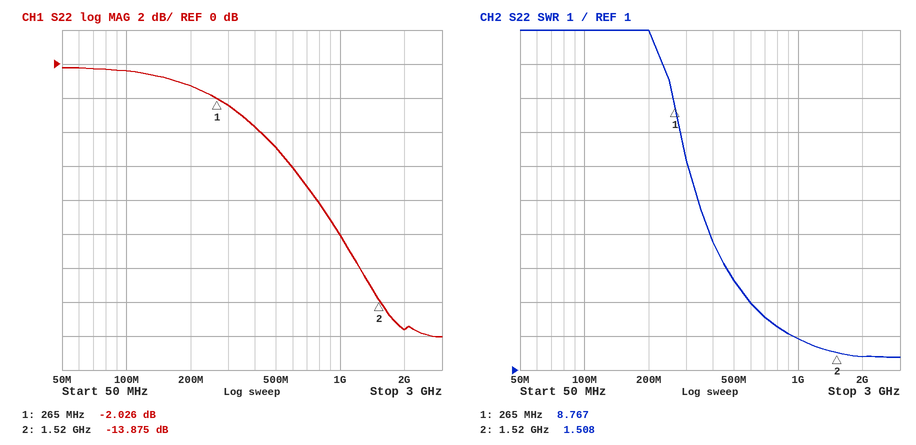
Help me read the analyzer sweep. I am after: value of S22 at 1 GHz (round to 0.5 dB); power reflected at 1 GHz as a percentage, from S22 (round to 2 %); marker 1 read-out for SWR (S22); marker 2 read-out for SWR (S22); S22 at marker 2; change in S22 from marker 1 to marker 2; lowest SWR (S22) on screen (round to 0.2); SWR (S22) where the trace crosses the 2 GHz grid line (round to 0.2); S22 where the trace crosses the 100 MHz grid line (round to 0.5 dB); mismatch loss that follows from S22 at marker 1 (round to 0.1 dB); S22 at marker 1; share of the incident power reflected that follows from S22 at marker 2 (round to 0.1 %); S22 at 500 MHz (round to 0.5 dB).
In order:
-10.0 dB
10 %
8.767
1.508
-13.875 dB
-11.849 dB
1.4
1.4
-0.5 dB
4.3 dB
-2.026 dB
4.1 %
-5.0 dB
